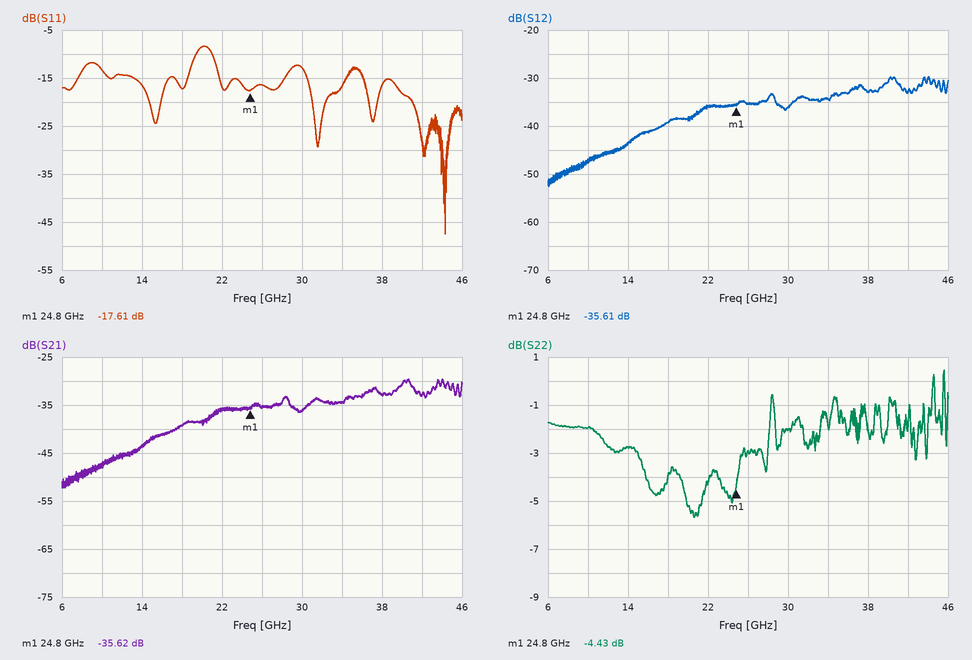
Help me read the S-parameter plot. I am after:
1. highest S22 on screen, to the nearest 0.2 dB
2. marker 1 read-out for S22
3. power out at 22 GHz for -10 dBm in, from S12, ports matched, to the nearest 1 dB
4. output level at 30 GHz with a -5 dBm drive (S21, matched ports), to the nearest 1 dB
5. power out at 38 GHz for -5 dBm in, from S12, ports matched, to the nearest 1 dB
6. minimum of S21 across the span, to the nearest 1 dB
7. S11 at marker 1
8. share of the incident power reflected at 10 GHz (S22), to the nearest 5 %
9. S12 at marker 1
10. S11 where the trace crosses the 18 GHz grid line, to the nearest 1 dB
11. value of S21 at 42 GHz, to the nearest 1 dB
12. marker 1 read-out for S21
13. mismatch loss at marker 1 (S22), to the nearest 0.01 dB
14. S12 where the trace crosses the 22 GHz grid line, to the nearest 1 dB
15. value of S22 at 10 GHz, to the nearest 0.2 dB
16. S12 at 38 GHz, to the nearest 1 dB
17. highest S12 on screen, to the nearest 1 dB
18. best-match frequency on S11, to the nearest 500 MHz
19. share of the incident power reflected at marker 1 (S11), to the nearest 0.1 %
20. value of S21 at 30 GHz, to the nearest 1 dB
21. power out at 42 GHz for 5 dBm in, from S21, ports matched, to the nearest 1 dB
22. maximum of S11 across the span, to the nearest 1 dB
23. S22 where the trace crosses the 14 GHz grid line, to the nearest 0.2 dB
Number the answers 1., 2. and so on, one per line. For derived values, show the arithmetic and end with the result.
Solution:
1. 0.4 dB
2. -4.43 dB
3. -10 dBm + (-36 dB) = -46 dBm
4. -5 dBm + (-36 dB) = -41 dBm
5. -5 dBm + (-33 dB) = -38 dBm
6. -52 dB
7. -17.61 dB
8. 10^(-2/10) ≈ 63.1 %, so 65 % to the nearest 5 %
9. -35.61 dB
10. -17 dB
11. -33 dB
12. -35.62 dB
13. −10 log10(1 − 10^(-4.43/10)) ≈ 1.94 dB
14. -36 dB
15. -2.0 dB
16. -33 dB
17. -30 dB
18. 44.5 GHz
19. 10^(-17.61/10) ≈ 1.7 %
20. -36 dB
21. 5 dBm + (-33 dB) = -28 dBm
22. -8 dB
23. -2.8 dB
